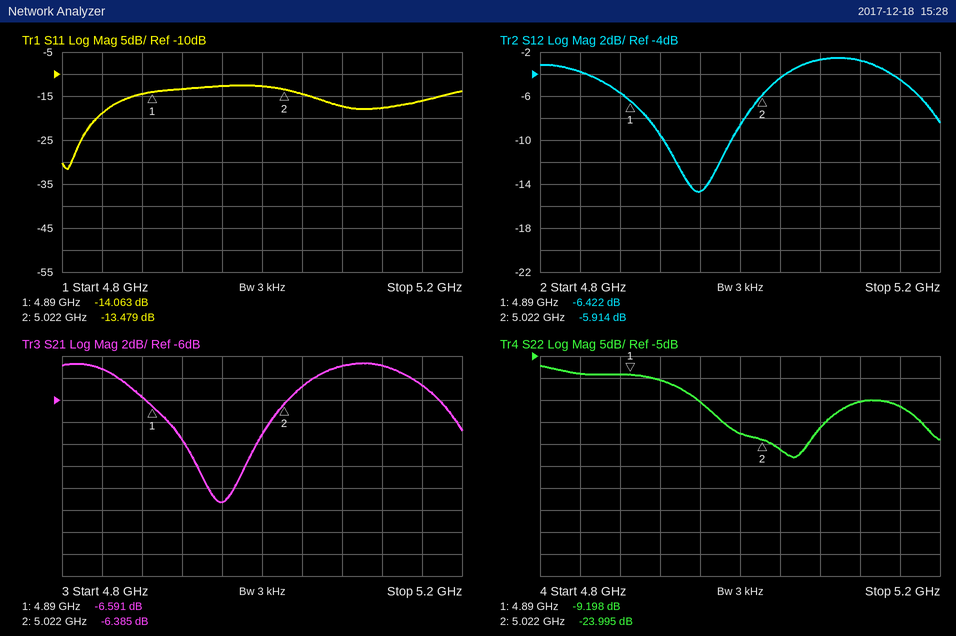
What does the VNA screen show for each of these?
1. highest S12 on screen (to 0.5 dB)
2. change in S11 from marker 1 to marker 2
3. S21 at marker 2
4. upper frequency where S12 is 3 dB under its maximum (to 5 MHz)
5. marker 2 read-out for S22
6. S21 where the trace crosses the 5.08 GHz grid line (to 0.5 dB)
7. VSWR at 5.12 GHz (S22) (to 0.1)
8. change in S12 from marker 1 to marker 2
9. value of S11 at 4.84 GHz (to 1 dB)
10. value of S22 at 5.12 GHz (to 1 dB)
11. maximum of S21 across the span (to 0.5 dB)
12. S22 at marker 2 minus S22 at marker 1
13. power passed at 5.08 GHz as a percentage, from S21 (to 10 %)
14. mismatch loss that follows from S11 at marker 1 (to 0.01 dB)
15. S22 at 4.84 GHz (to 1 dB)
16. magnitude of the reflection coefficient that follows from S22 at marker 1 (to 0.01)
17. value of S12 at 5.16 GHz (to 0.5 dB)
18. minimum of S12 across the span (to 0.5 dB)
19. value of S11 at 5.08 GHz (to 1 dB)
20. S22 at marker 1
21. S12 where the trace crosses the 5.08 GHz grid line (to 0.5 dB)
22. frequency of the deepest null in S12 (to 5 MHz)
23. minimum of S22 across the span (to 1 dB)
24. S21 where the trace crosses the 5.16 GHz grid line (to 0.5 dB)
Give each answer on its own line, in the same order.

-2.5 dB
0.584 dB
-6.385 dB
5.175 GHz
-23.995 dB
-3.0 dB
1.4
0.508 dB
-19 dB
-15 dB
-2.5 dB
-14.797 dB
50 %
0.17 dB
-9 dB
0.35
-4.5 dB
-14.5 dB
-17 dB
-9.198 dB
-2.5 dB
4.960 GHz
-28 dB
-4.5 dB
